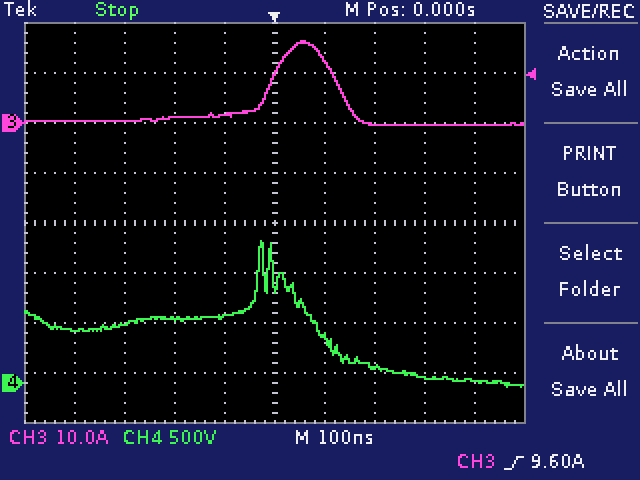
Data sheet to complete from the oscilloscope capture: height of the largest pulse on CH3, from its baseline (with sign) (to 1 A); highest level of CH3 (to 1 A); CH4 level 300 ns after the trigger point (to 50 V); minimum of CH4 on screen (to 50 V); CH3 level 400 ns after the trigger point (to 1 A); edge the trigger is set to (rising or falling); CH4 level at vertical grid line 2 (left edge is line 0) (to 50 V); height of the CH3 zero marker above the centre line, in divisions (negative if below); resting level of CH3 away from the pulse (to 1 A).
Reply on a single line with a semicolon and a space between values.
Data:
+16 A; 16 A; 50 V; -50 V; 0 A; rising; 600 V; +2.0 div; 0 A
